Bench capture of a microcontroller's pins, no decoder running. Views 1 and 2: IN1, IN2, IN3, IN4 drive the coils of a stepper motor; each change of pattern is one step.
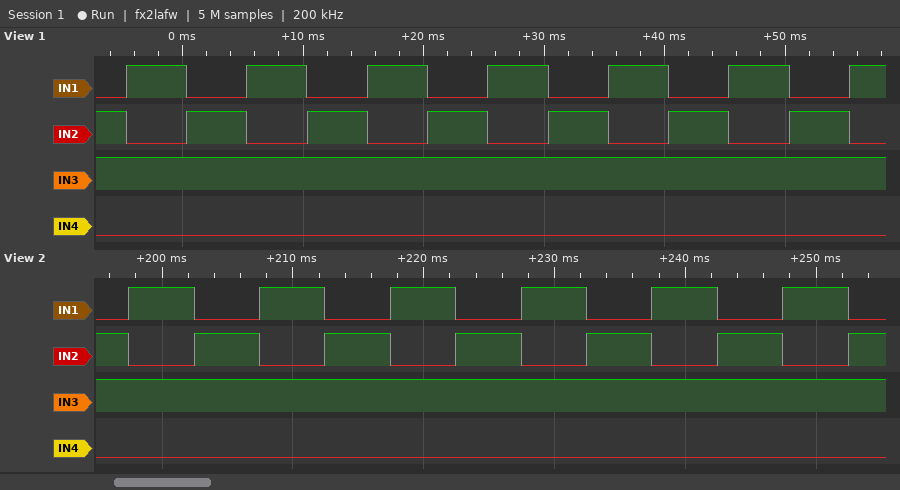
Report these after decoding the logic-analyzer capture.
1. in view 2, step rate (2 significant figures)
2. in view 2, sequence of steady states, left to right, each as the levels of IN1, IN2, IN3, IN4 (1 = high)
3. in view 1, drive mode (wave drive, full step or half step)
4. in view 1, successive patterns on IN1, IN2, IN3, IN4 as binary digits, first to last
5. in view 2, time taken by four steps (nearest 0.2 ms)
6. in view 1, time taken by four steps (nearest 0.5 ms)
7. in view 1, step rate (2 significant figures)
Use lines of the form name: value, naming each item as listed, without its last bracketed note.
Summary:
in view 2, step rate: 200 steps/s
in view 2, sequence of steady states, left to right, each as the levels of IN1, IN2, IN3, IN4: 0110 1010 0110 1010 0110 1010 0110 1010 0110 1010 0110 1010 0110
in view 1, drive mode: full step
in view 1, successive patterns on IN1, IN2, IN3, IN4 as binary digits, first to last: 0110 1010 0110 1010 0110 1010 0110 1010 0110 1010 0110 1010 0110 1010
in view 2, time taken by four steps: 20.0 ms
in view 1, time taken by four steps: 20.0 ms
in view 1, step rate: 200 steps/s
